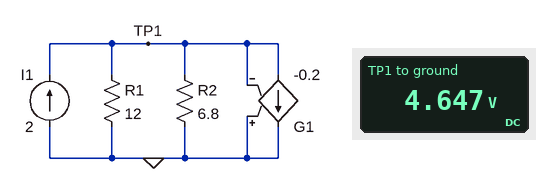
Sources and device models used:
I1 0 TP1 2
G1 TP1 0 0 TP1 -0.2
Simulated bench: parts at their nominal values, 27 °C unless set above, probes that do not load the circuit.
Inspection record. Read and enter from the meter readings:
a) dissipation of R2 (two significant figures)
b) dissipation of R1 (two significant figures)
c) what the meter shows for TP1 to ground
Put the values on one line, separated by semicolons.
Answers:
3.2 W; 1.8 W; 4.647 V
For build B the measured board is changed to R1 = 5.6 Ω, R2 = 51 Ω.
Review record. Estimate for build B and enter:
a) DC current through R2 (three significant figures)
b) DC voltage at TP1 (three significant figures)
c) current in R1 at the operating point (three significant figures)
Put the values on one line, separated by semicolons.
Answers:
98.5 mA; 5.02 V; 897 mA
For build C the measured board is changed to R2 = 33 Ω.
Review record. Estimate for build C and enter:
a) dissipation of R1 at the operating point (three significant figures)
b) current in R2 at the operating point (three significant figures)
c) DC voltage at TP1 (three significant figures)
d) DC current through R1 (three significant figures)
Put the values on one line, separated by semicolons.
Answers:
3.39 W; 193 mA; 6.38 V; 531 mA
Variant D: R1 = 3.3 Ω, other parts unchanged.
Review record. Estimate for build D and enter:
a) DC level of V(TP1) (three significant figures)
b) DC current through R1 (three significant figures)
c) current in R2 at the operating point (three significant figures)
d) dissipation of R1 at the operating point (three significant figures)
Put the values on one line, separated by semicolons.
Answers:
3.08 V; 932 mA; 452 mA; 2.87 W
